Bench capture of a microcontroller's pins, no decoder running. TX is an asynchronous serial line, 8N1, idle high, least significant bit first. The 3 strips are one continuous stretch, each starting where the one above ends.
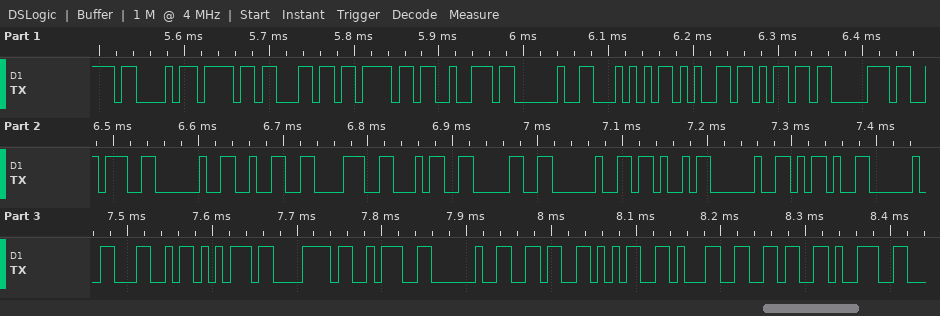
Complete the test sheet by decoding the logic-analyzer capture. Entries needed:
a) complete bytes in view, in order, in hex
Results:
43 6F 6C 6F 72 20 54 65 6D 70 3A 20 32 38 34 30 20 4B 20 2D 20 4C 75 78 3A 20 36 35 31 36 39
